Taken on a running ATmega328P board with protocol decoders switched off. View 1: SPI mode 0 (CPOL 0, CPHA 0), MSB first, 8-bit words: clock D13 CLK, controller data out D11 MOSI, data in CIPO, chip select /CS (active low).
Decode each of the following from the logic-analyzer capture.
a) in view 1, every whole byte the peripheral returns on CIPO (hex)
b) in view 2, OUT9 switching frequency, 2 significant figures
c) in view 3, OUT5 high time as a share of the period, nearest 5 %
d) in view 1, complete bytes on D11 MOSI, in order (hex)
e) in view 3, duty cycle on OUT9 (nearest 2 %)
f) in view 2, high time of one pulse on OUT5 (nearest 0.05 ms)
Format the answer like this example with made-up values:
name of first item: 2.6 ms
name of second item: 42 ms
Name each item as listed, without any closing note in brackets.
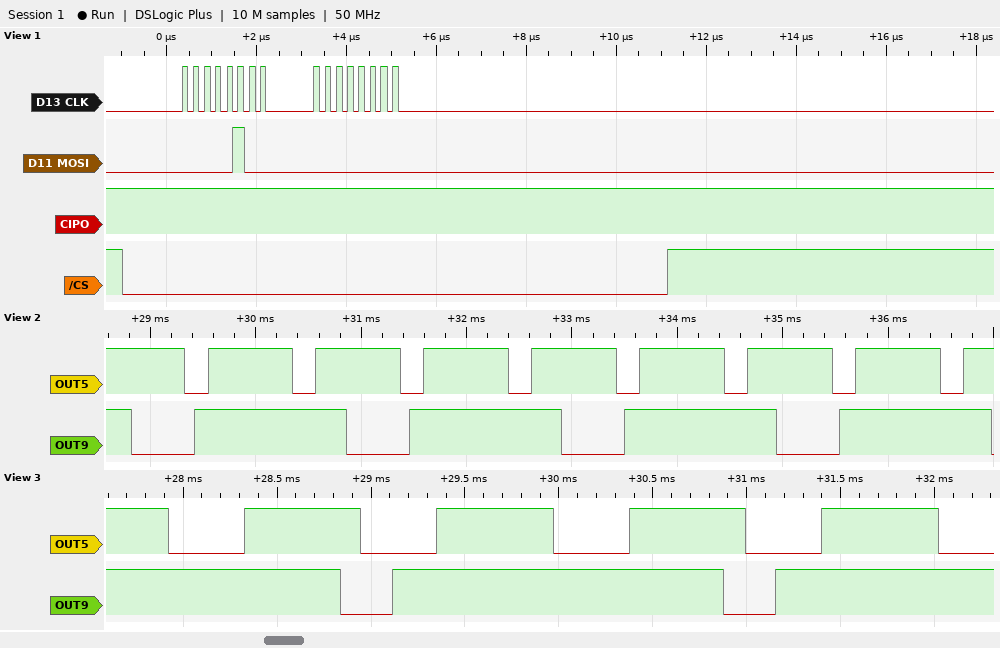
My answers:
in view 1, every whole byte the peripheral returns on CIPO: FF FF
in view 2, OUT9 switching frequency, 2 significant figures: 490 Hz
in view 3, OUT5 high time as a share of the period, nearest 5 %: 60 %
in view 1, complete bytes on D11 MOSI, in order: 04 00
in view 3, duty cycle on OUT9: 86 %
in view 2, high time of one pulse on OUT5: 0.80 ms
